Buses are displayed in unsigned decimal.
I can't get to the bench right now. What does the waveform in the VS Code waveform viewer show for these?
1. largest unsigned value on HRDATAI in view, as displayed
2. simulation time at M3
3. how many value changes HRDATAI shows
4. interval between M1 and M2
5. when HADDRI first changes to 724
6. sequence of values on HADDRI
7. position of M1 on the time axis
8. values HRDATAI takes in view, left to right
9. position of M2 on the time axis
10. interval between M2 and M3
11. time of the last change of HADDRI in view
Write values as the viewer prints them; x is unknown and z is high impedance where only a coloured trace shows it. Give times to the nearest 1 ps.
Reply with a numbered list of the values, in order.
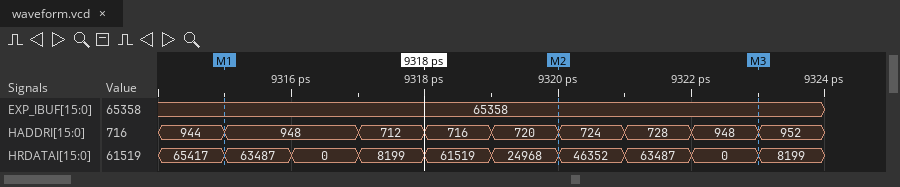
1. 65417
2. 9323 ps
3. 9
4. 5 ps
5. 9320 ps
6. 944, 948, 712, 716, 720, 724, 728, 948, 952
7. 9315 ps
8. 65417, 63487, 0, 8199, 61519, 24968, 46352, 63487, 0, 8199
9. 9320 ps
10. 3 ps
11. 9323 ps
